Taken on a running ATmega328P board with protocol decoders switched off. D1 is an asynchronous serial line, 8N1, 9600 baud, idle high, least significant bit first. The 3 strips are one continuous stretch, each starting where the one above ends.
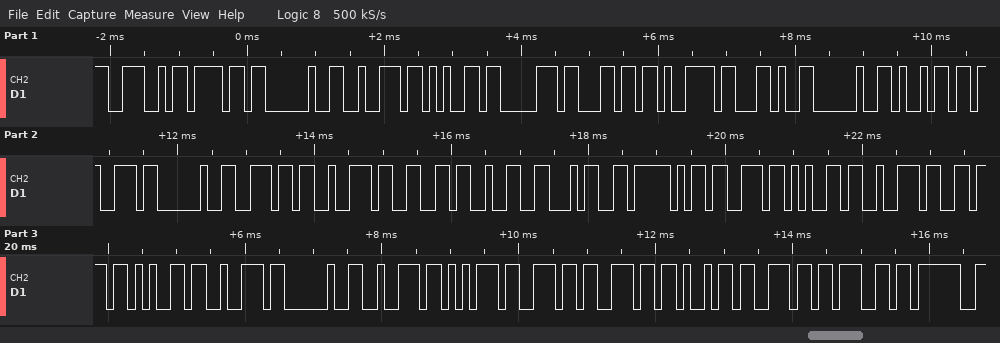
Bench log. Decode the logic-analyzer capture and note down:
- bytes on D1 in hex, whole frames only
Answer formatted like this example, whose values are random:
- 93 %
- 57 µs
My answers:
- 4E 6F 20 72 65 70 6C 79 2C 20 69 73 20 6E 72 66 32 34 5F 73 65 72 76 65 72 20 72 75 6E 6E 69 6E 67 3F
